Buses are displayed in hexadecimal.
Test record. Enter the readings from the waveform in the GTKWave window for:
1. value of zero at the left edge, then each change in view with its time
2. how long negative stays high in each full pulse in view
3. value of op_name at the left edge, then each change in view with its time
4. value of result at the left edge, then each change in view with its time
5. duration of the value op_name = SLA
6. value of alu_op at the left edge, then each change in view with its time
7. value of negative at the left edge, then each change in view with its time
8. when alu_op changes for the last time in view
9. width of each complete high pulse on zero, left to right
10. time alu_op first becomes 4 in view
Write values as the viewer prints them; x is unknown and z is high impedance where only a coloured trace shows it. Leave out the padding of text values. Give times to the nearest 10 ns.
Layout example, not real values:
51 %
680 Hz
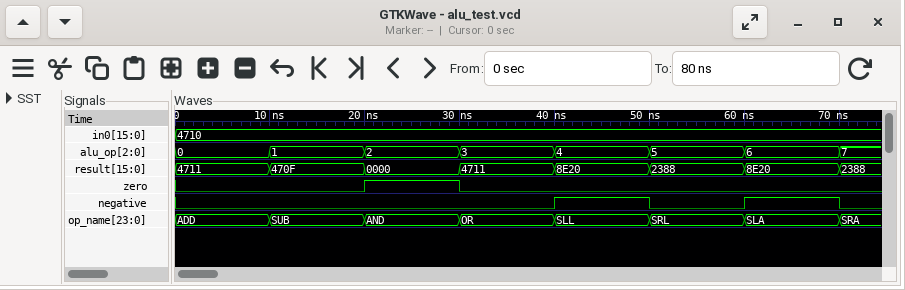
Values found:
0, 1 at 20 ns, 0 at 30 ns
10 ns, 10 ns
ADD, SUB at 10 ns, AND at 20 ns, OR at 30 ns, SLL at 40 ns, SRL at 50 ns, SLA at 60 ns, SRA at 70 ns
4711, 470F at 10 ns, 0000 at 20 ns, 4711 at 30 ns, 8E20 at 40 ns, 2388 at 50 ns, 8E20 at 60 ns, 2388 at 70 ns
10 ns
0, 1 at 10 ns, 2 at 20 ns, 3 at 30 ns, 4 at 40 ns, 5 at 50 ns, 6 at 60 ns, 7 at 70 ns
0, 1 at 40 ns, 0 at 50 ns, 1 at 60 ns, 0 at 70 ns
70 ns
10 ns
40 ns
